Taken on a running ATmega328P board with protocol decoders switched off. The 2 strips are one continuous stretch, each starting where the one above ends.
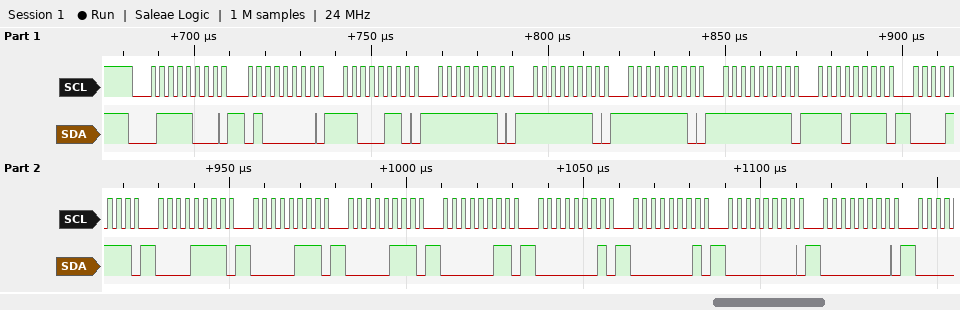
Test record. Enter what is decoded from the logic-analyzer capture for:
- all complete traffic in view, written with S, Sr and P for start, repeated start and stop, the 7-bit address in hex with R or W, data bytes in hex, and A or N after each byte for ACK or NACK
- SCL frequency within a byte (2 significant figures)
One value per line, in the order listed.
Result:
S 3CW A 40 A C6 A FE A FE A FE A FF A EF A 0F A 0F A 07 A 07 A 03 A 01 A 01 A 00 A 00 A
400 kHz
